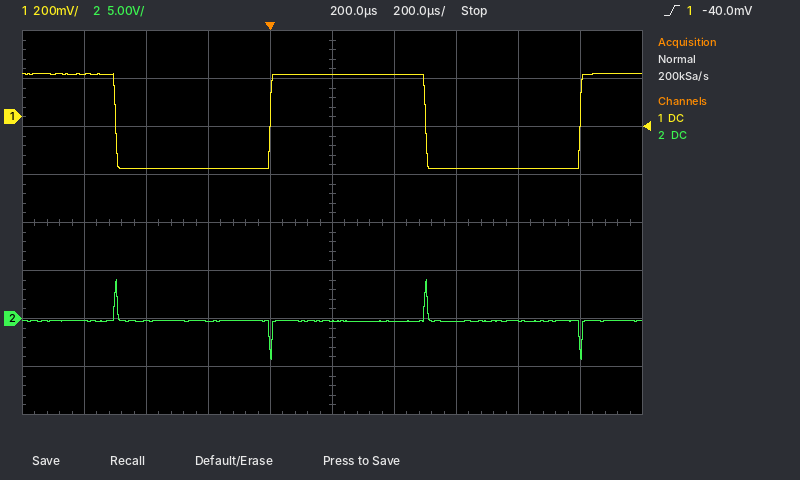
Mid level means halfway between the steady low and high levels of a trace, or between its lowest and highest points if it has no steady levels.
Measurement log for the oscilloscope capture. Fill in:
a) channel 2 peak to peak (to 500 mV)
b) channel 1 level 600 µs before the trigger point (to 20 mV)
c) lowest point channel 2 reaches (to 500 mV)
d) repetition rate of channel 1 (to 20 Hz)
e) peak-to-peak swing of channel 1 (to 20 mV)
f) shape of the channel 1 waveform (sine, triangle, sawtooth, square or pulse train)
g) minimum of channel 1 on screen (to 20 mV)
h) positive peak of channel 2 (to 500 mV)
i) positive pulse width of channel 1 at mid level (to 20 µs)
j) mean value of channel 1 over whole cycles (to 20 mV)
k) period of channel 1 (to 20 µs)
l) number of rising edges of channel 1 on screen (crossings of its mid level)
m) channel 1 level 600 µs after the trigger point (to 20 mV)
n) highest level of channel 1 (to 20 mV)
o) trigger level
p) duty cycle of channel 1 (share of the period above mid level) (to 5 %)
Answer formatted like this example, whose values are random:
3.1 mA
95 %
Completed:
8.5 V
180 mV
-4.5 V
1.00 kHz
400 mV
square
-220 mV
4.0 V
500 µs
-20 mV
1.00 ms
2
-220 mV
180 mV
-40.0 mV
50 %
